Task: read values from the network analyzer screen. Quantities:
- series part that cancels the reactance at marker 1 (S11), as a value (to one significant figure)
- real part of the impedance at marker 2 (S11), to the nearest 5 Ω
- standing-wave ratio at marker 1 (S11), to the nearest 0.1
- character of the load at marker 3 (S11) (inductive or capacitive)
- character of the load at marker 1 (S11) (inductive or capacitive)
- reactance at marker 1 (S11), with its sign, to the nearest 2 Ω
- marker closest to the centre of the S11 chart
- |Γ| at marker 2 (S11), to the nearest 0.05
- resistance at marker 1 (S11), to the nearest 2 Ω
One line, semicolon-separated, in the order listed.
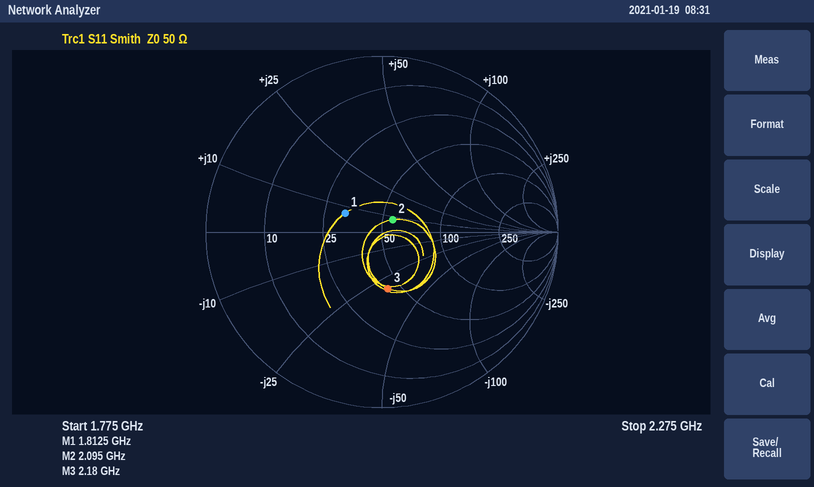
10 pF; 55 Ω; 1.6; capacitive; inductive; +8 Ω; marker 2; 0.10; 32 Ω
